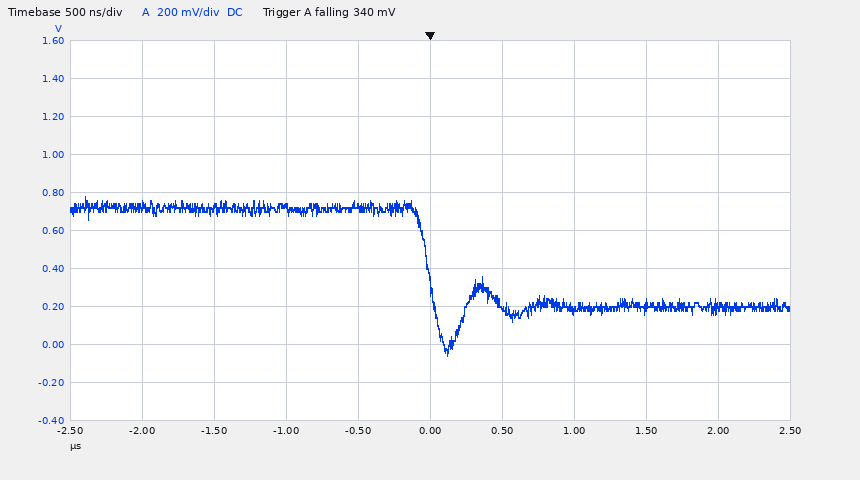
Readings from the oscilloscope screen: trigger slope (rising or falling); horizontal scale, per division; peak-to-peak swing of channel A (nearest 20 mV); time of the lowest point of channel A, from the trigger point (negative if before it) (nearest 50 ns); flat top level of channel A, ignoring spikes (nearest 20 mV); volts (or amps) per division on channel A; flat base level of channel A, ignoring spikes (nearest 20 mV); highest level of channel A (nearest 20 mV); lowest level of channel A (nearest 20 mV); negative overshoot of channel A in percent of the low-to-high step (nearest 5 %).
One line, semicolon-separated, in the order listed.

falling; 500 ns; 840 mV; +100 ns; 720 mV; 200 mV; 200 mV; 780 mV; -60 mV; 50 %
